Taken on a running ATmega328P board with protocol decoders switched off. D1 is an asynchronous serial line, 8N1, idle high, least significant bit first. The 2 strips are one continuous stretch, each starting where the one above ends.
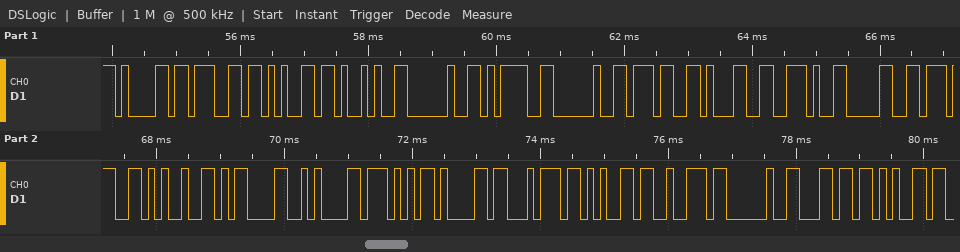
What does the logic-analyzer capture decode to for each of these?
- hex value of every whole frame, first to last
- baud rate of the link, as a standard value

61 67 65 29 20 3D 20 37 31 2E 30 37 25 0D 0A 57 61 74 65 72 20 6C 65
9600 baud
